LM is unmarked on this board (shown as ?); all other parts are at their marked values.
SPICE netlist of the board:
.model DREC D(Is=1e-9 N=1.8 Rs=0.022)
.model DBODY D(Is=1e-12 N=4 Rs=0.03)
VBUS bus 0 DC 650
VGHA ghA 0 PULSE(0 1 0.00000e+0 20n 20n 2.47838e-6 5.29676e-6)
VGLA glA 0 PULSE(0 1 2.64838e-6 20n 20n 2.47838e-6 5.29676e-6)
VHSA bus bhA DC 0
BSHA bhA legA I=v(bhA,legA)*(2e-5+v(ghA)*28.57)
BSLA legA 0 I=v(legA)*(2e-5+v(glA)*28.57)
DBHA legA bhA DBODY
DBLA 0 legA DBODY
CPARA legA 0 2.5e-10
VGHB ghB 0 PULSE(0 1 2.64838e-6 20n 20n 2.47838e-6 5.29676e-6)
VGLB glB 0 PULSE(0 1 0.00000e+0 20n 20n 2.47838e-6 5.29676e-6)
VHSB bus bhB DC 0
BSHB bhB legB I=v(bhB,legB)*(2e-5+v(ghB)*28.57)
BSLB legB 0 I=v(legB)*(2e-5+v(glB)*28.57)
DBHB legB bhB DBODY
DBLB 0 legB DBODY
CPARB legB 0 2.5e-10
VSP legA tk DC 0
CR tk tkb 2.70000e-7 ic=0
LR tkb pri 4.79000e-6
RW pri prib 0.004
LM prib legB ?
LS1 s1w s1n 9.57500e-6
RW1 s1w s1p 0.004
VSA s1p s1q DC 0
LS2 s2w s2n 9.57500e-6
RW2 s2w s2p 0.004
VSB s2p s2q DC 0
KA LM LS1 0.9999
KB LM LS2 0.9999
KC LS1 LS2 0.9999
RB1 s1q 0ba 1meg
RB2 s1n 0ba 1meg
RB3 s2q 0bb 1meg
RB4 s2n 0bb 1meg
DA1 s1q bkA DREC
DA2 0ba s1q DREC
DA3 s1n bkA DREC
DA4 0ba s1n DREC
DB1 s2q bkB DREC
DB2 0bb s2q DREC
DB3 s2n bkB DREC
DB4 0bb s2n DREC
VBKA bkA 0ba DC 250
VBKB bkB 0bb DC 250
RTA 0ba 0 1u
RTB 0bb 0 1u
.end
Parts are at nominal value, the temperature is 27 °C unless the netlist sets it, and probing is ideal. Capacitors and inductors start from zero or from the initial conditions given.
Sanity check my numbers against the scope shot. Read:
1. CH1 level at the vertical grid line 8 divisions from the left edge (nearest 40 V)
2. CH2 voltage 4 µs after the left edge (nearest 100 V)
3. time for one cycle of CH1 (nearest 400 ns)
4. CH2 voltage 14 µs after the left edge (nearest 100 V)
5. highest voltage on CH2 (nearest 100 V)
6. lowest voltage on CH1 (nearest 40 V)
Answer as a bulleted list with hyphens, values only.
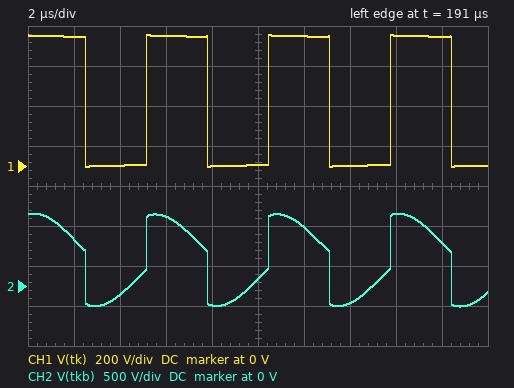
- 640 V
- -100 V
- 5.2 µs
- -200 V
- 900 V
- 0 V
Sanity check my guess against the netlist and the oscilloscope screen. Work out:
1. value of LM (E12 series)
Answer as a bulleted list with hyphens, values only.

- 47 µH
